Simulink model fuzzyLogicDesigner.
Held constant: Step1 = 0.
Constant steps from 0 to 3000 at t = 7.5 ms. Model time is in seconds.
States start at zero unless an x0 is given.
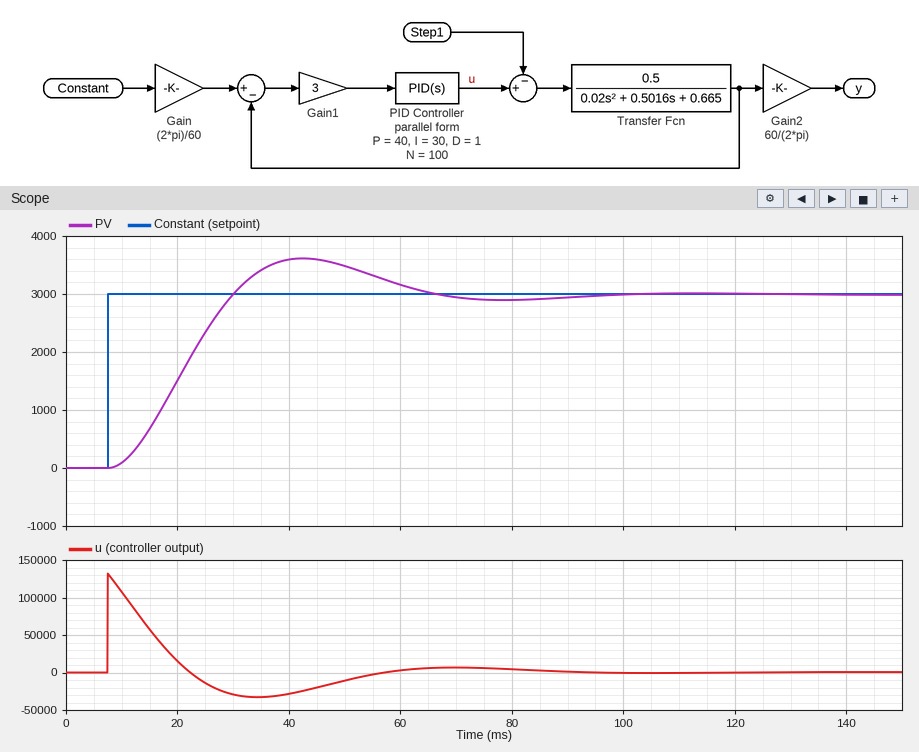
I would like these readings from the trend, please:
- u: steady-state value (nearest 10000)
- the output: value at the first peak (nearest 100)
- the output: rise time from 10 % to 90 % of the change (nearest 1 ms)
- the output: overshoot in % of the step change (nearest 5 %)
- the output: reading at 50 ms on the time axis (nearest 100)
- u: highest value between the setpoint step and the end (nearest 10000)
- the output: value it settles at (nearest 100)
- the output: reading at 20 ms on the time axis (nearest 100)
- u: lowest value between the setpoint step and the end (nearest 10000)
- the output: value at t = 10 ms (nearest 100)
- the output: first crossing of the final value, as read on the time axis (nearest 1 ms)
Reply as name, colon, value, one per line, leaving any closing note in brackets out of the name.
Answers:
u: steady-state value: 0
the output: value at the first peak: 3600
the output: rise time from 10 % to 90 % of the change: 15 ms
the output: overshoot in % of the step change: 20 %
the output: reading at 50 ms on the time axis: 3500
u: highest value between the setpoint step and the end: 130000
the output: value it settles at: 3000
the output: reading at 20 ms on the time axis: 1500
u: lowest value between the setpoint step and the end: -30000
the output: value at t = 10 ms: 100
the output: first crossing of the final value, as read on the time axis: 30 ms
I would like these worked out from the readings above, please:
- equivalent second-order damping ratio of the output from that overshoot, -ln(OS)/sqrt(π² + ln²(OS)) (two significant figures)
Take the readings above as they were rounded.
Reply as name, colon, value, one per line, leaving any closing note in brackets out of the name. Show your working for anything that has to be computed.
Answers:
equivalent second-order damping ratio of the output from that overshoot, -ln(OS)/sqrt(π² + ln²(OS)): ln(0.2) = -1.609; 1.609 / sqrt(9.870 + 2.590) = 0.46
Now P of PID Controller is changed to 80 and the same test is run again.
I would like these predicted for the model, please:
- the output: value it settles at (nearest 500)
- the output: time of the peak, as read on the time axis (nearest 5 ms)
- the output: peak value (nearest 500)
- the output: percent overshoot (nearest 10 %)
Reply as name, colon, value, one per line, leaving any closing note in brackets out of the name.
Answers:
the output: value it settles at: 3000
the output: time of the peak, as read on the time axis: 35 ms
the output: peak value: 4000
the output: percent overshoot: 40 %
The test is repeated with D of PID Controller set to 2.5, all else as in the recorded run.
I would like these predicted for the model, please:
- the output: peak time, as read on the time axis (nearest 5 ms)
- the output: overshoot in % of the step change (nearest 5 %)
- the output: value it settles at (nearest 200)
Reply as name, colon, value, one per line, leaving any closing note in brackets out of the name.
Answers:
the output: peak time, as read on the time axis: 30 ms
the output: overshoot in % of the step change: 25 %
the output: value it settles at: 3000
